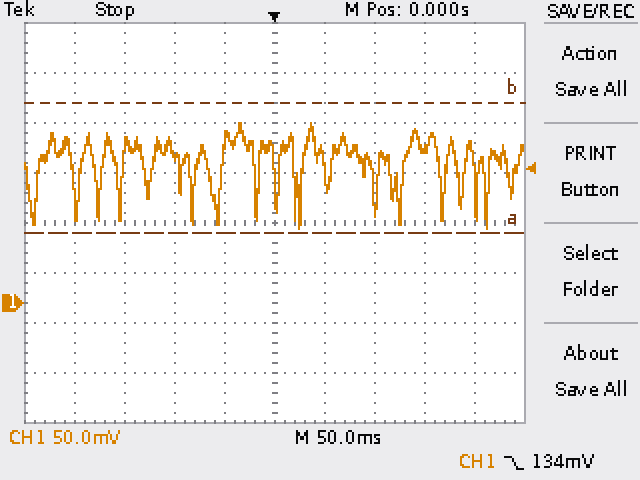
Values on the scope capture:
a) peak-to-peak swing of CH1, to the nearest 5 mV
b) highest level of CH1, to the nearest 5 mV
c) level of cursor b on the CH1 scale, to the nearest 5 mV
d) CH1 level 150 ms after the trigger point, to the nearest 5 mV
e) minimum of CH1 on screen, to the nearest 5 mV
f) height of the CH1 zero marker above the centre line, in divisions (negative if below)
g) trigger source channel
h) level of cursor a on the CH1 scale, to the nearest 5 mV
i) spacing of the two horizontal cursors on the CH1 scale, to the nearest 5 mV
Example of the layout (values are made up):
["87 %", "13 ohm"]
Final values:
["105 mV", "180 mV", "200 mV", "155 mV", "75 mV", "-1.6 div", "CH1", "70 mV", "130 mV"]
